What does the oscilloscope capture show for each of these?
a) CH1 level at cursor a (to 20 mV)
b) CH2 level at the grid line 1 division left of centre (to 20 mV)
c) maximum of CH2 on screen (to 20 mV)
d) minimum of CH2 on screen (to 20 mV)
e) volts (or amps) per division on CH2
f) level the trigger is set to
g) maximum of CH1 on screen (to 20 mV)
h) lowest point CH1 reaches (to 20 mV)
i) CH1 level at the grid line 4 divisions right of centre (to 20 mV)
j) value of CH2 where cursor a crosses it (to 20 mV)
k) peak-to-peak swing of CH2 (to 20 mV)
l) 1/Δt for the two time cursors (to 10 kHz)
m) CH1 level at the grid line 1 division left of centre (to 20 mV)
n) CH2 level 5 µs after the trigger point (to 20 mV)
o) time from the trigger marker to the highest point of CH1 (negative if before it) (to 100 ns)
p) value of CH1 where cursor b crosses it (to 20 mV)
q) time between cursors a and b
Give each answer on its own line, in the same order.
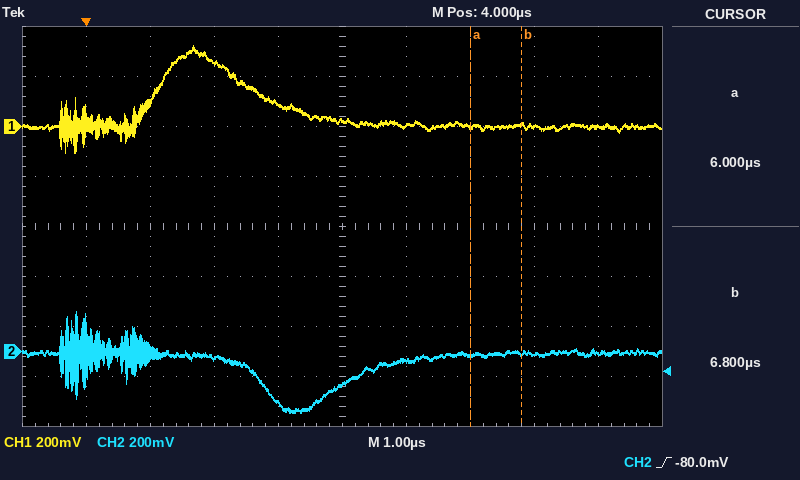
0 mV
-200 mV
160 mV
-240 mV
200 mV
-80.0 mV
320 mV
-100 mV
0 mV
-20 mV
400 mV
1.25 MHz
100 mV
-40 mV
+1.7 µs
0 mV
800 ns
